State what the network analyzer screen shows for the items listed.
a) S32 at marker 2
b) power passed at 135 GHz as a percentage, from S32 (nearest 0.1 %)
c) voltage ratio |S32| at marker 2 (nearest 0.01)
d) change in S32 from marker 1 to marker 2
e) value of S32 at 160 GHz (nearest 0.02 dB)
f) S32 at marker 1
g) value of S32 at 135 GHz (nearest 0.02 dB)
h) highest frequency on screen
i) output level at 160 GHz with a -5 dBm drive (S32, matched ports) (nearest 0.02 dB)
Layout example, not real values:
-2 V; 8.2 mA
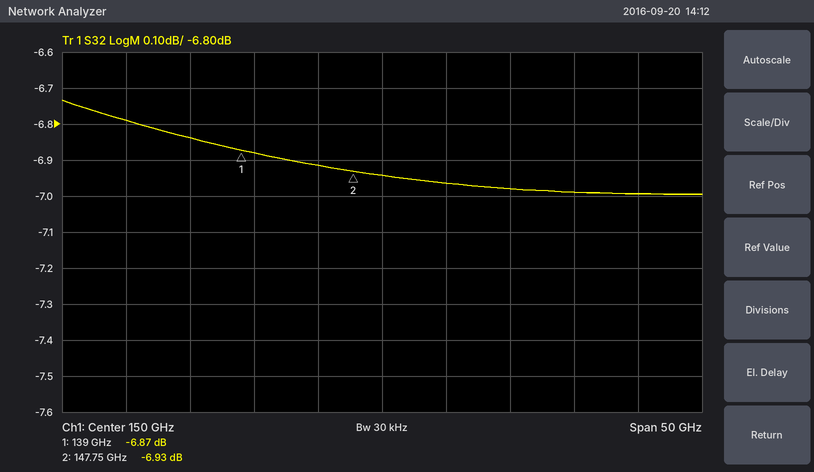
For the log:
-6.93 dB; 20.7 %; 0.45; -0.06 dB; -6.98 dB; -6.87 dB; -6.84 dB; 175 GHz; -11.98 dBm
